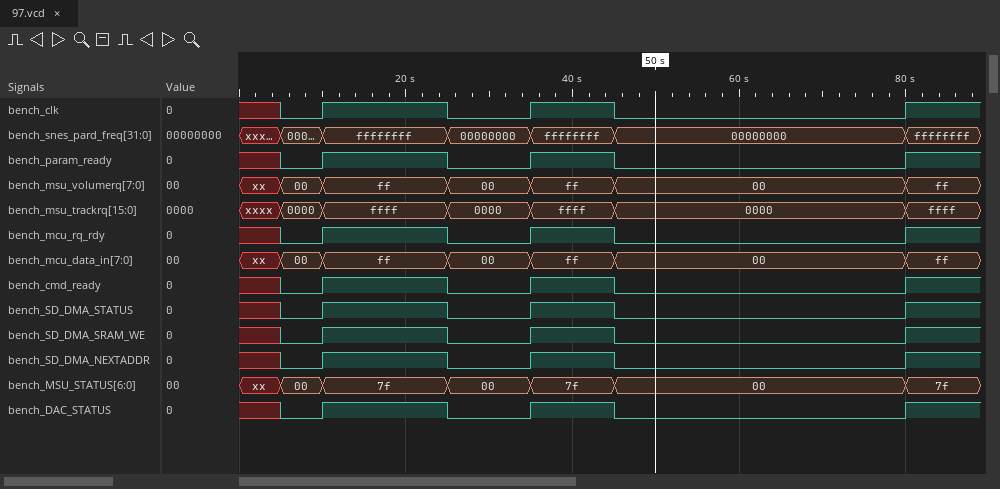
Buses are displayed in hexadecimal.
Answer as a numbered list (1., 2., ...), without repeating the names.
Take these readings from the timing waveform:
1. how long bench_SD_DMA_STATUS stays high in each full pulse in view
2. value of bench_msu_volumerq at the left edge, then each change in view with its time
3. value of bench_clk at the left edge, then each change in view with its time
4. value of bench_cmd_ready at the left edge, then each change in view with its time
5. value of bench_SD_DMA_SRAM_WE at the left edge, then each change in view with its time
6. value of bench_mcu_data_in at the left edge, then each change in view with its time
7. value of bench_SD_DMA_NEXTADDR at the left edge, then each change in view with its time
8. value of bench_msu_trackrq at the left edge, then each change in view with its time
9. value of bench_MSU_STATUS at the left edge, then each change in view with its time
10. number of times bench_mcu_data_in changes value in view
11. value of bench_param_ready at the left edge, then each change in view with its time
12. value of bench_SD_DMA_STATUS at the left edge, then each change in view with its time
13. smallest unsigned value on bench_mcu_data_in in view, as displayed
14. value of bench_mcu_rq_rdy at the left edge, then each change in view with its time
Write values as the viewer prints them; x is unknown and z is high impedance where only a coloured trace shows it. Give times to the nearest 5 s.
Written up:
1. 15 s, 10 s
2. xx, 00 at 5 s, ff at 10 s, 00 at 25 s, ff at 35 s, 00 at 45 s, ff at 80 s
3. x, 0 at 5 s, 1 at 10 s, 0 at 25 s, 1 at 35 s, 0 at 45 s, 1 at 80 s
4. x, 0 at 5 s, 1 at 10 s, 0 at 25 s, 1 at 35 s, 0 at 45 s, 1 at 80 s
5. x, 0 at 5 s, 1 at 10 s, 0 at 25 s, 1 at 35 s, 0 at 45 s, 1 at 80 s
6. xx, 00 at 5 s, ff at 10 s, 00 at 25 s, ff at 35 s, 00 at 45 s, ff at 80 s
7. x, 0 at 5 s, 1 at 10 s, 0 at 25 s, 1 at 35 s, 0 at 45 s, 1 at 80 s
8. xxxx, 0000 at 5 s, ffff at 10 s, 0000 at 25 s, ffff at 35 s, 0000 at 45 s, ffff at 80 s
9. xx, 00 at 5 s, 7f at 10 s, 00 at 25 s, 7f at 35 s, 00 at 45 s, 7f at 80 s
10. 6
11. x, 0 at 5 s, 1 at 10 s, 0 at 25 s, 1 at 35 s, 0 at 45 s, 1 at 80 s
12. x, 0 at 5 s, 1 at 10 s, 0 at 25 s, 1 at 35 s, 0 at 45 s, 1 at 80 s
13. 00
14. x, 0 at 5 s, 1 at 10 s, 0 at 25 s, 1 at 35 s, 0 at 45 s, 1 at 80 s
